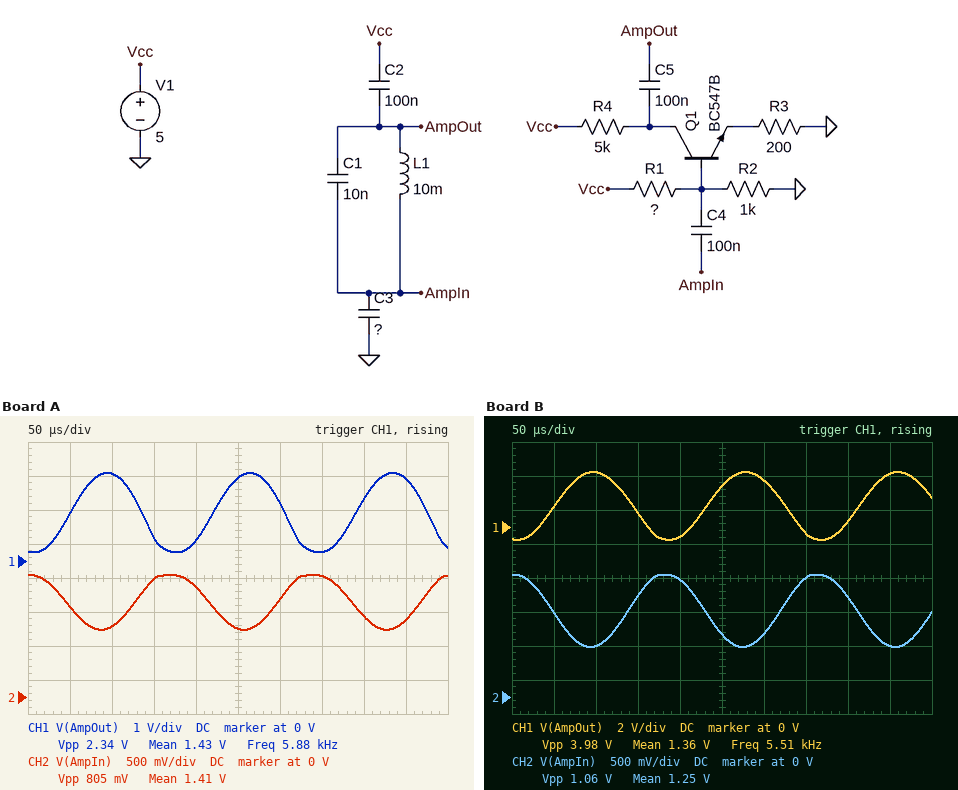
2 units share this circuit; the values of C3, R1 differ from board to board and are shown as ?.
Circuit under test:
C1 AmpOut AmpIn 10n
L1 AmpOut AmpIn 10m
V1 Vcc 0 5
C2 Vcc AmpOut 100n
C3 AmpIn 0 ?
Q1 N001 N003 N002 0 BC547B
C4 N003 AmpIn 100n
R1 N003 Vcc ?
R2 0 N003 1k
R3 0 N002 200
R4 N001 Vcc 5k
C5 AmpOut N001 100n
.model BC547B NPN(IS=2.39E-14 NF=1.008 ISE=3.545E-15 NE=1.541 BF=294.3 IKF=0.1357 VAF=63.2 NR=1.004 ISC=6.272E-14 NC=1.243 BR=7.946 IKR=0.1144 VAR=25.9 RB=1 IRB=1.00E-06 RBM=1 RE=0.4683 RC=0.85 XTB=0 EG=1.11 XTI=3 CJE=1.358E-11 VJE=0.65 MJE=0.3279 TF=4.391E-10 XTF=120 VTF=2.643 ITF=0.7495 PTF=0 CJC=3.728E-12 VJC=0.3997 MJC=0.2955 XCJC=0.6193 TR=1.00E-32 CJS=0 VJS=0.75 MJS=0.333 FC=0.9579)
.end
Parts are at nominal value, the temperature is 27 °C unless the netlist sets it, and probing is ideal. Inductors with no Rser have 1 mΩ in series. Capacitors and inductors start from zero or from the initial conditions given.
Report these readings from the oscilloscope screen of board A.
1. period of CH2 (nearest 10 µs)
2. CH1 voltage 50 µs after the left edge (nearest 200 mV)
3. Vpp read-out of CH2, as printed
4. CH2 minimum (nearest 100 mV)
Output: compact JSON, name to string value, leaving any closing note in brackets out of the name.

{"period of CH2": "170 µs", "CH1 voltage 50 µs after the left edge": "1.4 V", "Vpp read-out of CH2, as printed": "805 mV", "CH2 minimum": "1.0 V"}
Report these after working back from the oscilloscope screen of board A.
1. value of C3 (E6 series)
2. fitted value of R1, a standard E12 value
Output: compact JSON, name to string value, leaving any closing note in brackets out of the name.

{"value of C3": "220 nF", "fitted value of R1, a standard E12 value": "4.7 kΩ"}
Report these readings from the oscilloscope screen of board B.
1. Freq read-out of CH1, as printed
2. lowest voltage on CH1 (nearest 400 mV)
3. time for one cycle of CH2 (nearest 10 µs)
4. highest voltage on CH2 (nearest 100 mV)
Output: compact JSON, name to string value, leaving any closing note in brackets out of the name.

{"Freq read-out of CH1, as printed": "5.51 kHz", "lowest voltage on CH1": "-800 mV", "time for one cycle of CH2": "180 µs", "highest voltage on CH2": "1.8 V"}
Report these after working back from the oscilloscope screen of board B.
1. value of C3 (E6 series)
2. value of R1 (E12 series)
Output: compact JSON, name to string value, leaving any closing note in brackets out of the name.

{"value of C3": "330 nF", "value of R1": "6.8 kΩ"}
